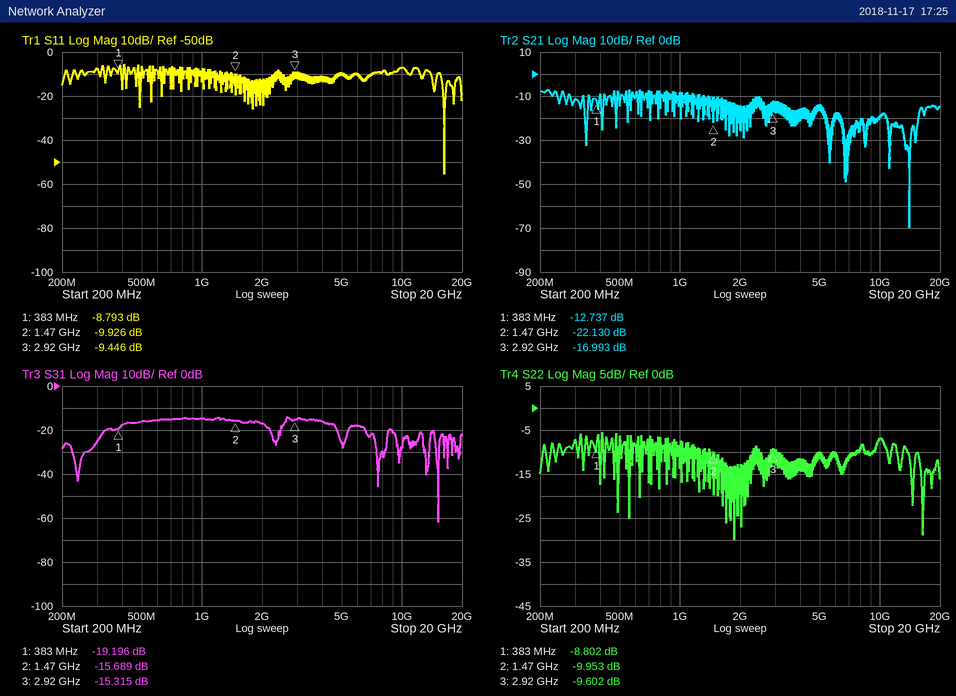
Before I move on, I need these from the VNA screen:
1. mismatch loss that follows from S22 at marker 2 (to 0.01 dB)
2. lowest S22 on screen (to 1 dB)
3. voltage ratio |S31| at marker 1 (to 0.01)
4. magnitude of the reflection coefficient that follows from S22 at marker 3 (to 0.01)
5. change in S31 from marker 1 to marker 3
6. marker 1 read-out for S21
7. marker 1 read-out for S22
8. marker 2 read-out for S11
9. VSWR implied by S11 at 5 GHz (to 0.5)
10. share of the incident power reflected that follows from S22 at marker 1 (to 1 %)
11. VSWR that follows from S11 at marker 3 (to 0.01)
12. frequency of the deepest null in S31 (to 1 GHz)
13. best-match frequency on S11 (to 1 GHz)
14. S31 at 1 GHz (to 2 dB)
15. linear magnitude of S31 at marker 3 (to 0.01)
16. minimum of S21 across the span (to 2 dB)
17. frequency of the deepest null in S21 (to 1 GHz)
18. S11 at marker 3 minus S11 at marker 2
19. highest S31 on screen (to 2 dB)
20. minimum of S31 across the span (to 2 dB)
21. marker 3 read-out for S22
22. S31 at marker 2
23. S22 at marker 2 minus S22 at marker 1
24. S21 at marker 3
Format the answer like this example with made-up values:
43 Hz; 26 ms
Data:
0.46 dB; -30 dB; 0.11; 0.33; 3.881 dB; -12.737 dB; -8.802 dB; -9.926 dB; 2.0; 13 %; 2.02; 15 GHz; 16 GHz; -14 dB; 0.17; -70 dB; 14 GHz; 0.480 dB; -14 dB; -62 dB; -9.602 dB; -15.689 dB; -1.151 dB; -16.993 dB
